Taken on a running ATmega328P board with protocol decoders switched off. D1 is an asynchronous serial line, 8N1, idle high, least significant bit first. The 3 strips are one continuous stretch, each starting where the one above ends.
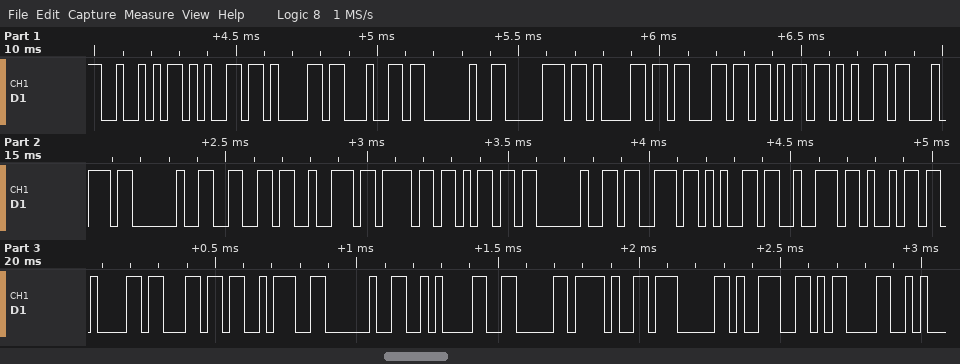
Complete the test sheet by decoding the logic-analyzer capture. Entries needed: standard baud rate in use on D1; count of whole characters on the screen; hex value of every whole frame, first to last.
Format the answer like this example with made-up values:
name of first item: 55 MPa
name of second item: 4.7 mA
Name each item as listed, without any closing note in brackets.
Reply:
standard baud rate in use on D1: 38400 baud
count of whole characters on the screen: 31
hex value of every whole frame, first to last: 0x52 0x65 0x61 0x64 0x20 0x70 0x61 0x63 0x6B 0x65 0x74 0x20 0x66 0x72 0x6F 0x6D 0x20 0x73 0x65 0x72 0x69 0x61 0x6C 0x3A 0x20 0x0A 0x06 0x2F 0x07 0x39 0x0D
